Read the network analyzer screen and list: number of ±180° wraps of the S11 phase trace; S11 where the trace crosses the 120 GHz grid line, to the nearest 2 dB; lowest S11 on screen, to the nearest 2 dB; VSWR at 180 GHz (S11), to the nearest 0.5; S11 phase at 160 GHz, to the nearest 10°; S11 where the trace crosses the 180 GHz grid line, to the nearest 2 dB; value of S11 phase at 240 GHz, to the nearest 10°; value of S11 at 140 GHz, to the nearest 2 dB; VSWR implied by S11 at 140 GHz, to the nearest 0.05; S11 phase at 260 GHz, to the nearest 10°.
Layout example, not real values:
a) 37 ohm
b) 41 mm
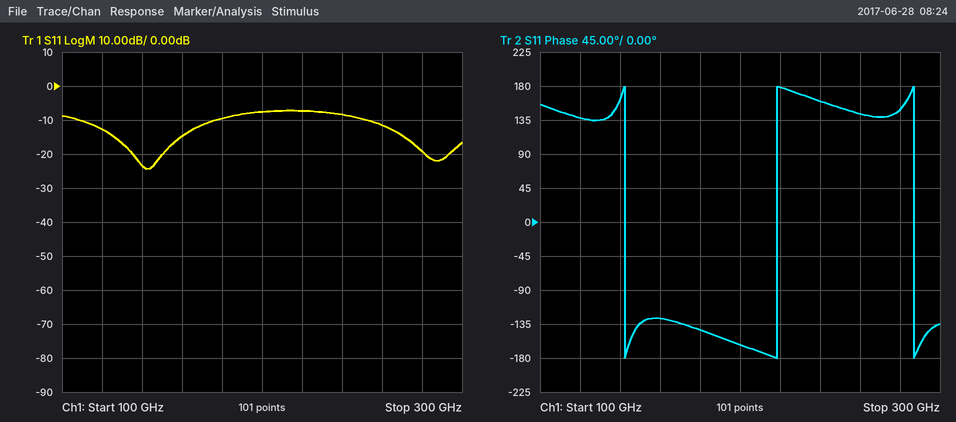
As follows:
a) 3
b) -12 dB
c) -24 dB
d) 2.0
e) -130°
f) -10 dB
g) 160°
h) -24 dB
i) 1.15
j) 140°
